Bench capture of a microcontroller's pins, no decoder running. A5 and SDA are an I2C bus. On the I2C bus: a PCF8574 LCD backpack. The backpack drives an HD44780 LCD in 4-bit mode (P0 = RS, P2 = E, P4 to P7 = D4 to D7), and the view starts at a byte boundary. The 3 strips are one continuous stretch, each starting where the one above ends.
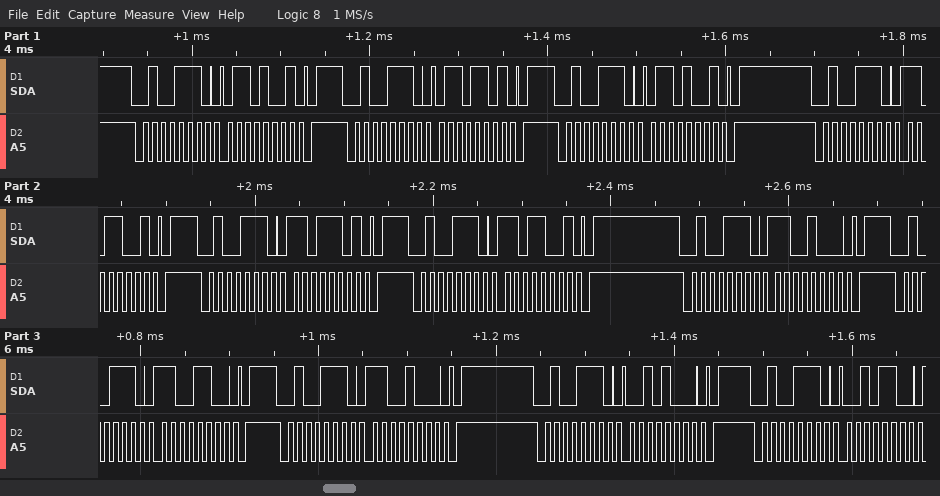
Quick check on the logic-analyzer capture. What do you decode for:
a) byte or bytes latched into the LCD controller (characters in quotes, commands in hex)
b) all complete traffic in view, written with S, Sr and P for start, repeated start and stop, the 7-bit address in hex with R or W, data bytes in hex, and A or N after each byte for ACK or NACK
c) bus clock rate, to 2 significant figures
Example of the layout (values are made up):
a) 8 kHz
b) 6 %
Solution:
a) 'm'
b) S 27W A 69 A P S 27W A 6D A P S 27W A 69 A P S 27W A D9 A P S 27W A DD A P S 27W A D9 A P S 27W A C8 A P S 27W A CC A P S 27W A C8 A P S 27W A 28 A P S 27W A 2C A
c) 100 kHz
